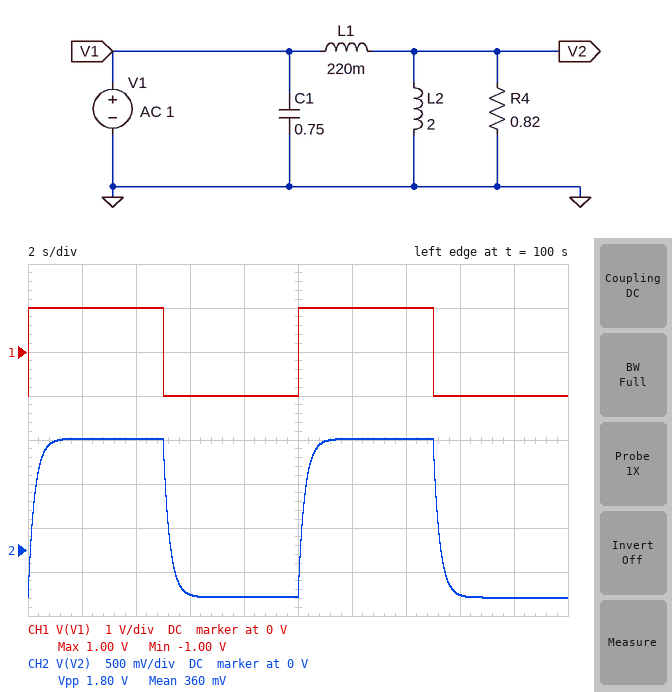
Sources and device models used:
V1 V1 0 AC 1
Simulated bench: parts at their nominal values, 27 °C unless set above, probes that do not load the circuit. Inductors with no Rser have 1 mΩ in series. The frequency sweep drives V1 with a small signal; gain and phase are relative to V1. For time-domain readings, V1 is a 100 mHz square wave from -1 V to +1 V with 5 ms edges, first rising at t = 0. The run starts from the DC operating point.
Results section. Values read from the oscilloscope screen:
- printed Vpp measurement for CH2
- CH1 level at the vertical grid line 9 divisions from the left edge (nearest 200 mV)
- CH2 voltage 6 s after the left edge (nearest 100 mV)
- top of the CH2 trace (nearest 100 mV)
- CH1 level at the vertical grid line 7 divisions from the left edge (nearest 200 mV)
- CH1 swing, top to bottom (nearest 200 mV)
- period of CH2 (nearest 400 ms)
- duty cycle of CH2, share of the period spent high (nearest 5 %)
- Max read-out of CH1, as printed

1.80 V
-1.0 V
-500 mV
1.3 V
1.0 V
2.0 V
10.0 s
50 %
1.00 V
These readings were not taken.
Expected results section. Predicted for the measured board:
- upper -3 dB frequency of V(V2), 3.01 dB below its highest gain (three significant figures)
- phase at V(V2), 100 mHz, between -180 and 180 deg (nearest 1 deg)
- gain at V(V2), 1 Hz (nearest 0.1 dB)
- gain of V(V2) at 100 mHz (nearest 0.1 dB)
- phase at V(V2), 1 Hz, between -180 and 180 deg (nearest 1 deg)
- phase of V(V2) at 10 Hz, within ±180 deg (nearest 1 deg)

659 mHz
-9 deg
-6.1 dB
-1.0 dB
-57 deg
-86 deg
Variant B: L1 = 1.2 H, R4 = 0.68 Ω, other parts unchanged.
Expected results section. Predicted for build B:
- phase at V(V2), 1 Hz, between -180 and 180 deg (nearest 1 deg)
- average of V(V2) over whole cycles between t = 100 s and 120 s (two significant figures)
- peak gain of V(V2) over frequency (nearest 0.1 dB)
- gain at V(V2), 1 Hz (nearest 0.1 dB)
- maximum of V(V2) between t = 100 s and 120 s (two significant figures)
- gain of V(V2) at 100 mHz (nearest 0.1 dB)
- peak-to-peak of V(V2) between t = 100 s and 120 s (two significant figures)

-82 deg
120 mV
-4.1 dB
-21.0 dB
730 mV
-5.8 dB
1.2 V
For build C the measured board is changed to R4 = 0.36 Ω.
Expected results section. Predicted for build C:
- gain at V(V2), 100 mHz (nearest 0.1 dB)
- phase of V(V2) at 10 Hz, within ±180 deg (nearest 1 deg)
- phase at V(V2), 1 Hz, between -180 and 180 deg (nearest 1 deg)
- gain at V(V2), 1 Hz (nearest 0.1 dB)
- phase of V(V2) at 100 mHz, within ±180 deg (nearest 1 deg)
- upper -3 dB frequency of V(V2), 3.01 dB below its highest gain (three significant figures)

-1.4 dB
-88 deg
-74 deg
-12.0 dB
-19 deg
290 mHz
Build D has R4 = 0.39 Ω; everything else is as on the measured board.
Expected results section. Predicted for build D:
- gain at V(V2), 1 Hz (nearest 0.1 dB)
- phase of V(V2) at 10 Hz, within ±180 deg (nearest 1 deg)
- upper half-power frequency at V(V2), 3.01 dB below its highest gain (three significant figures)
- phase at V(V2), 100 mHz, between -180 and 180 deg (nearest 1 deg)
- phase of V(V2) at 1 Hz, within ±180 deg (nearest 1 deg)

-11.4 dB
-88 deg
314 mHz
-18 deg
-73 deg
